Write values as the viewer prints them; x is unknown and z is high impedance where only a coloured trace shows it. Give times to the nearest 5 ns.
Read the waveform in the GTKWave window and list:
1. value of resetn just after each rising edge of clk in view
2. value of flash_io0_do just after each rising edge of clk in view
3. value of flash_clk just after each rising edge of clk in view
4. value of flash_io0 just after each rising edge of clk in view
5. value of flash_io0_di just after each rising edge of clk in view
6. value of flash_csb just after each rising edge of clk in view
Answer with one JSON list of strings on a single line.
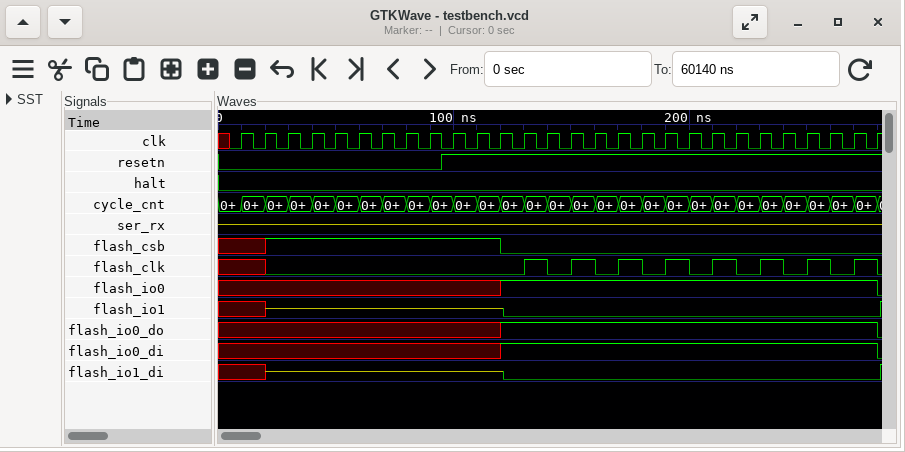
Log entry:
["0 0 0 0 0 0 0 0 0 1 1 1 1 1 1 1 1 1 1 1 1 1 1 1 1 1 1 1", "x x x x x x x x x x x 1 1 1 1 1 1 1 1 1 1 1 1 1 1 1 1 0", "x 0 0 0 0 0 0 0 0 0 0 0 1 0 1 0 1 0 1 0 1 0 1 0 1 0 1 0", "x x x x x x x x x x x 1 1 1 1 1 1 1 1 1 1 1 1 1 1 1 1 0", "x x x x x x x x x x x 1 1 1 1 1 1 1 1 1 1 1 1 1 1 1 1 0", "x 1 1 1 1 1 1 1 1 1 1 0 0 0 0 0 0 0 0 0 0 0 0 0 0 0 0 0"]
